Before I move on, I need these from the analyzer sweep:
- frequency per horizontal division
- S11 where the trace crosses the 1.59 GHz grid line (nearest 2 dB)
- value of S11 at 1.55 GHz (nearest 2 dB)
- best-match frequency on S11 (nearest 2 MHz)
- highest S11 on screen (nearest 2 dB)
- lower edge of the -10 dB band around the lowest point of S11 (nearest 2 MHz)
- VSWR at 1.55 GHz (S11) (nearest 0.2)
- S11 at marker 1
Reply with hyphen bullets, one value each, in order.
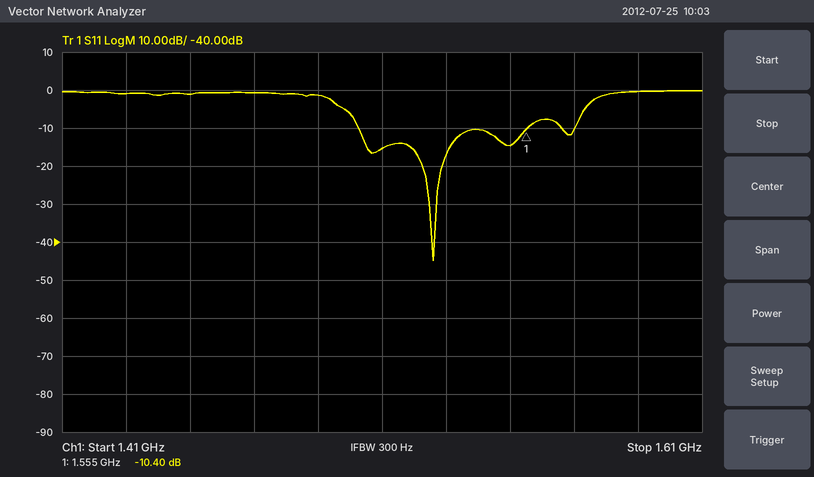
- 20 MHz
- 0 dB
- -14 dB
- 1.526 GHz
- 0 dB
- 1.502 GHz
- 1.4
- -10.40 dB
